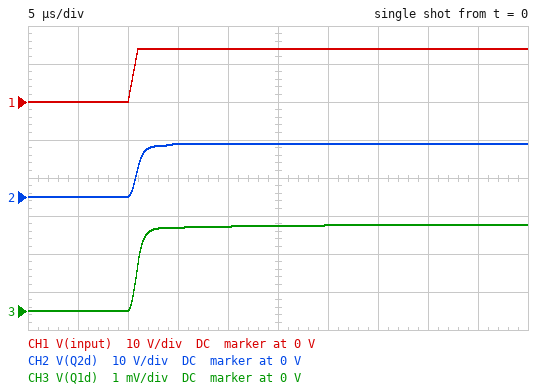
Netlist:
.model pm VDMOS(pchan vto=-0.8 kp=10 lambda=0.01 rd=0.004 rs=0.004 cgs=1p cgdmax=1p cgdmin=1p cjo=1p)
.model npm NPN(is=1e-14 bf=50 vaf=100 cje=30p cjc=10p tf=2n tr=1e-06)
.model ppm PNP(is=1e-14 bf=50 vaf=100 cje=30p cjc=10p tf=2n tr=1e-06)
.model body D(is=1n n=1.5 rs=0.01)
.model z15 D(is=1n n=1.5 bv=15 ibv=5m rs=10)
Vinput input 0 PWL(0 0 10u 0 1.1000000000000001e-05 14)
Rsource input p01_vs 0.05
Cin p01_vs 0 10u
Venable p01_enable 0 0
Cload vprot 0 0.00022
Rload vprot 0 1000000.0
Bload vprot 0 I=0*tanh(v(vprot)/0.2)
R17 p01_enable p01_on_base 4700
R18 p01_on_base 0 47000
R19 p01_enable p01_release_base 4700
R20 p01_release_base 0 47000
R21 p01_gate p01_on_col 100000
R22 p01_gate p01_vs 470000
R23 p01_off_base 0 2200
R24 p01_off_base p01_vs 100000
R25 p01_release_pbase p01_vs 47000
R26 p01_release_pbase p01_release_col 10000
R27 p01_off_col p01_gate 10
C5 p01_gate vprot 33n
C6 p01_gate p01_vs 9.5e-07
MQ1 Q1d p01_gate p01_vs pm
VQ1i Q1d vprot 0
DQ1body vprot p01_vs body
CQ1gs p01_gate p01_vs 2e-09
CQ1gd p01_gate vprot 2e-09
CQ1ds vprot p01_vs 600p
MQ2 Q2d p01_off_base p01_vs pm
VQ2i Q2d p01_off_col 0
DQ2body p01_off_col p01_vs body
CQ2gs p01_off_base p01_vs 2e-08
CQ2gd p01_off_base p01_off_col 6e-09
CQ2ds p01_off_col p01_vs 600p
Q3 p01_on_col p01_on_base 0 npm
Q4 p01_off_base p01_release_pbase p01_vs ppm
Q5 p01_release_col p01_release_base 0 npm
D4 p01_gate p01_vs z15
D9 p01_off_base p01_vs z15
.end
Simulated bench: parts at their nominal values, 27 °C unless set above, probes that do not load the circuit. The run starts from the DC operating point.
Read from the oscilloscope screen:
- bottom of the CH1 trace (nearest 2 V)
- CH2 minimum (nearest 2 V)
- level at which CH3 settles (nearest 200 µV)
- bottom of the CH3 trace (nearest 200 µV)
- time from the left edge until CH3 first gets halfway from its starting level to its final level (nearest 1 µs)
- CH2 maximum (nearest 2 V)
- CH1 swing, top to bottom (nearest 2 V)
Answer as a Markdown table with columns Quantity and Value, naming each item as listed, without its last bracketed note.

| Quantity | Value |
|---|---|
| bottom of the CH1 trace | 0 V |
| CH2 minimum | 0 V |
| level at which CH3 settles | 2.2 mV |
| bottom of the CH3 trace | 0 V |
| time from the left edge until CH3 first gets halfway from its starting level to its final level | 11 µs |
| CH2 maximum | 14 V |
| CH1 swing, top to bottom | 14 V |
